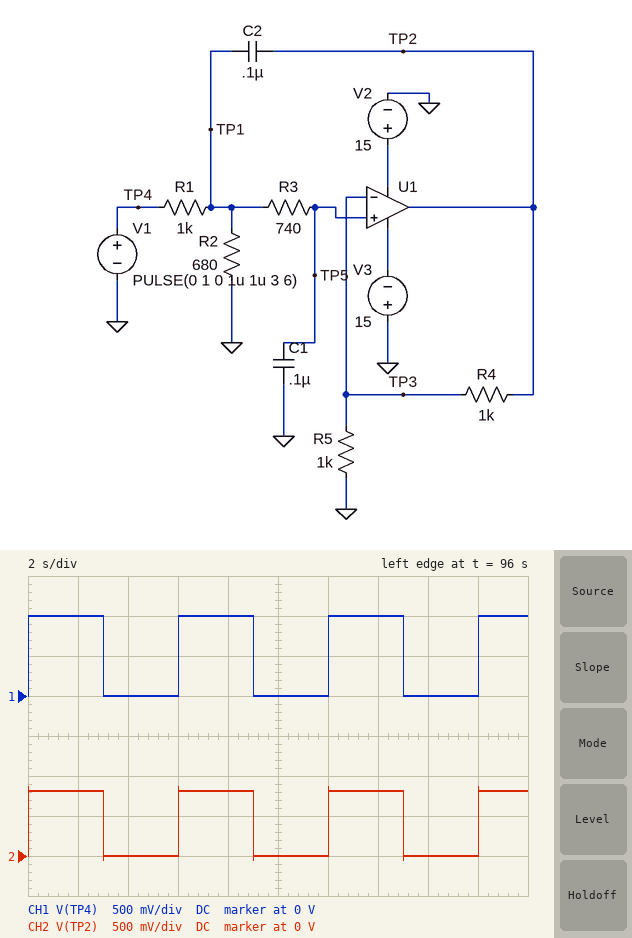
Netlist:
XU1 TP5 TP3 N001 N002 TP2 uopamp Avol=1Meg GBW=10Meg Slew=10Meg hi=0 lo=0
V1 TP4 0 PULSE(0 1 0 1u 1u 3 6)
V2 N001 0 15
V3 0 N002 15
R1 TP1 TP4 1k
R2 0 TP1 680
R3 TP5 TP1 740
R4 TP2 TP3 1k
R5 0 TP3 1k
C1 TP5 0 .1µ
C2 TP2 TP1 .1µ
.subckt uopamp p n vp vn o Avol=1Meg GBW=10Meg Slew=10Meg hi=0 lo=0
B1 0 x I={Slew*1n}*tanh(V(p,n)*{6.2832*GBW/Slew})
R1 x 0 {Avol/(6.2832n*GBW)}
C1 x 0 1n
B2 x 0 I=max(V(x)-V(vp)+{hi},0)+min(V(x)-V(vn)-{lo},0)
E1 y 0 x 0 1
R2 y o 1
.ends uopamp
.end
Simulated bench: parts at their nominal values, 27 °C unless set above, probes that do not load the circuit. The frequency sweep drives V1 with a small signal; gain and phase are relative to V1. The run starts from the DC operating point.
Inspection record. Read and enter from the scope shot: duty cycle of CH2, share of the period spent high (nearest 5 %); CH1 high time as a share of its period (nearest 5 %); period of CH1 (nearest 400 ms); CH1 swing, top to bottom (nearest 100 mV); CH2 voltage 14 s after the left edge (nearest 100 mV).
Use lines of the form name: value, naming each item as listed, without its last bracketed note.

duty cycle of CH2, share of the period spent high: 50 %
CH1 high time as a share of its period: 50 %
period of CH1: 6.0 s
CH1 swing, top to bottom: 1.0 V
CH2 voltage 14 s after the left edge: 800 mV
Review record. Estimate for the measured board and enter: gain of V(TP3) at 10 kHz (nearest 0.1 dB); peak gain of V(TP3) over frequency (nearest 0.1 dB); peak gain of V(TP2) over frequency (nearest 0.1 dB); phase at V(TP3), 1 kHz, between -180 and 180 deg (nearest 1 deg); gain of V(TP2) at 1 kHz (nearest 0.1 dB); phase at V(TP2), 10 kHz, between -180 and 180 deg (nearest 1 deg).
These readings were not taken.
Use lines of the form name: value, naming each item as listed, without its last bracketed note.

gain of V(TP3) at 10 kHz: -29.3 dB
peak gain of V(TP3) over frequency: -7.8 dB
peak gain of V(TP2) over frequency: -1.8 dB
phase at V(TP3), 1 kHz, between -180 and 180 deg: -28 deg
gain of V(TP2) at 1 kHz: -1.8 dB
phase at V(TP2), 10 kHz, between -180 and 180 deg: -157 deg
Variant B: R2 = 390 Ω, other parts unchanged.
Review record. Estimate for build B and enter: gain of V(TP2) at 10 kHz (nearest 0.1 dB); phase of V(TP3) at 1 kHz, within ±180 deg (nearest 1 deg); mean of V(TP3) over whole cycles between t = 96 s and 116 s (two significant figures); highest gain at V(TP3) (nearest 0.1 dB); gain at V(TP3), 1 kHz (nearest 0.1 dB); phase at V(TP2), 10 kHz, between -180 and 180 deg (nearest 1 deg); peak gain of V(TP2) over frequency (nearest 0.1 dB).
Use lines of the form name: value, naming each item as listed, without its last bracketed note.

gain of V(TP2) at 10 kHz: -23.7 dB
phase of V(TP3) at 1 kHz, within ±180 deg: -27 deg
mean of V(TP3) over whole cycles between t = 96 s and 116 s: 140 mV
highest gain at V(TP3): -11.0 dB
gain at V(TP3), 1 kHz: -11.3 dB
phase at V(TP2), 10 kHz, between -180 and 180 deg: -147 deg
peak gain of V(TP2) over frequency: -5.0 dB
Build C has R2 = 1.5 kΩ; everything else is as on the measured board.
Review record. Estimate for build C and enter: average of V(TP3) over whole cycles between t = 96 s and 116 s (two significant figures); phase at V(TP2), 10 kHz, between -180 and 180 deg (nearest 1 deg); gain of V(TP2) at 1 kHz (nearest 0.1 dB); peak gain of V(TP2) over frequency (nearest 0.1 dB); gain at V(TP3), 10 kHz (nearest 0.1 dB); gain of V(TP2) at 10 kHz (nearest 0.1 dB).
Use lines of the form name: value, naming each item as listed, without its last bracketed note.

average of V(TP3) over whole cycles between t = 96 s and 116 s: 300 mV
phase at V(TP2), 10 kHz, between -180 and 180 deg: -164 deg
gain of V(TP2) at 1 kHz: 2.1 dB
peak gain of V(TP2) over frequency: 2.3 dB
gain at V(TP3), 10 kHz: -29.1 dB
gain of V(TP2) at 10 kHz: -23.1 dB
